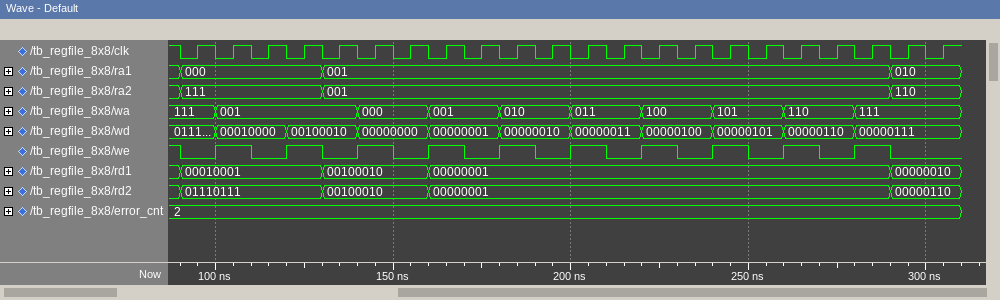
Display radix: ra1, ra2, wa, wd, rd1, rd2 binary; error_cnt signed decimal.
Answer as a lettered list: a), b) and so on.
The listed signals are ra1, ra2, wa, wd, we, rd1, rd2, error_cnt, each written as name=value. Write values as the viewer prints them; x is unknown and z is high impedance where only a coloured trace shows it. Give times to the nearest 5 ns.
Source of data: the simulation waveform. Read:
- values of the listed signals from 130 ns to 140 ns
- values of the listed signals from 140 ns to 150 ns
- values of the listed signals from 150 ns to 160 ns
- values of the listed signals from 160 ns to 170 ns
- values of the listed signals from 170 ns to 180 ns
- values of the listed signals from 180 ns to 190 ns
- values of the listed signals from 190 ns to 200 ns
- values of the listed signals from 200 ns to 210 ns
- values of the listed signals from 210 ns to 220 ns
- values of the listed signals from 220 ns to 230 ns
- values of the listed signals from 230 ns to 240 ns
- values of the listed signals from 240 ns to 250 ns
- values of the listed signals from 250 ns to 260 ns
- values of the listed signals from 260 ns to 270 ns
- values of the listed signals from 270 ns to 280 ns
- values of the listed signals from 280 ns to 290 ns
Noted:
a) ra1=001, ra2=001, wa=001, wd=00100010, we=0, rd1=00100010, rd2=00100010, error_cnt=2
b) ra1=001, ra2=001, wa=000, wd=00000000, we=1, rd1=00100010, rd2=00100010, error_cnt=2
c) ra1=001, ra2=001, wa=000, wd=00000000, we=0, rd1=00100010, rd2=00100010, error_cnt=2
d) ra1=001, ra2=001, wa=001, wd=00000001, we=1, rd1=00000001, rd2=00000001, error_cnt=2
e) ra1=001, ra2=001, wa=001, wd=00000001, we=0, rd1=00000001, rd2=00000001, error_cnt=2
f) ra1=001, ra2=001, wa=010, wd=00000010, we=1, rd1=00000001, rd2=00000001, error_cnt=2
g) ra1=001, ra2=001, wa=010, wd=00000010, we=0, rd1=00000001, rd2=00000001, error_cnt=2
h) ra1=001, ra2=001, wa=011, wd=00000011, we=1, rd1=00000001, rd2=00000001, error_cnt=2
i) ra1=001, ra2=001, wa=011, wd=00000011, we=0, rd1=00000001, rd2=00000001, error_cnt=2
j) ra1=001, ra2=001, wa=100, wd=00000100, we=1, rd1=00000001, rd2=00000001, error_cnt=2
k) ra1=001, ra2=001, wa=100, wd=00000100, we=0, rd1=00000001, rd2=00000001, error_cnt=2
l) ra1=001, ra2=001, wa=101, wd=00000101, we=1, rd1=00000001, rd2=00000001, error_cnt=2
m) ra1=001, ra2=001, wa=101, wd=00000101, we=0, rd1=00000001, rd2=00000001, error_cnt=2
n) ra1=001, ra2=001, wa=110, wd=00000110, we=1, rd1=00000001, rd2=00000001, error_cnt=2
o) ra1=001, ra2=001, wa=110, wd=00000110, we=0, rd1=00000001, rd2=00000001, error_cnt=2
p) ra1=001, ra2=001, wa=111, wd=00000111, we=1, rd1=00000001, rd2=00000001, error_cnt=2
